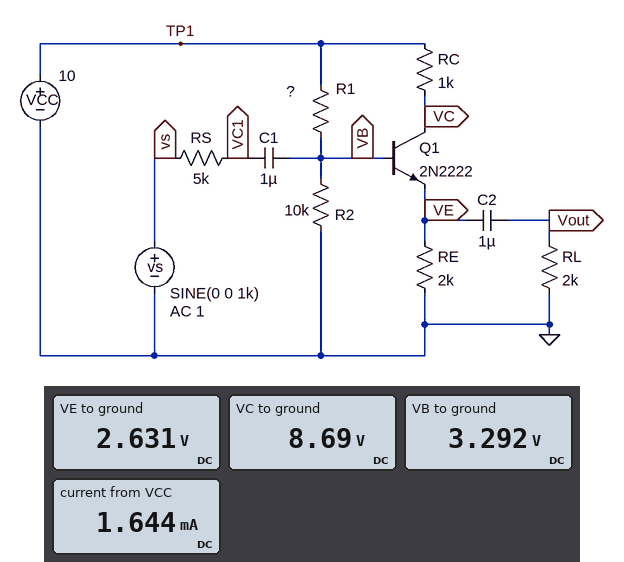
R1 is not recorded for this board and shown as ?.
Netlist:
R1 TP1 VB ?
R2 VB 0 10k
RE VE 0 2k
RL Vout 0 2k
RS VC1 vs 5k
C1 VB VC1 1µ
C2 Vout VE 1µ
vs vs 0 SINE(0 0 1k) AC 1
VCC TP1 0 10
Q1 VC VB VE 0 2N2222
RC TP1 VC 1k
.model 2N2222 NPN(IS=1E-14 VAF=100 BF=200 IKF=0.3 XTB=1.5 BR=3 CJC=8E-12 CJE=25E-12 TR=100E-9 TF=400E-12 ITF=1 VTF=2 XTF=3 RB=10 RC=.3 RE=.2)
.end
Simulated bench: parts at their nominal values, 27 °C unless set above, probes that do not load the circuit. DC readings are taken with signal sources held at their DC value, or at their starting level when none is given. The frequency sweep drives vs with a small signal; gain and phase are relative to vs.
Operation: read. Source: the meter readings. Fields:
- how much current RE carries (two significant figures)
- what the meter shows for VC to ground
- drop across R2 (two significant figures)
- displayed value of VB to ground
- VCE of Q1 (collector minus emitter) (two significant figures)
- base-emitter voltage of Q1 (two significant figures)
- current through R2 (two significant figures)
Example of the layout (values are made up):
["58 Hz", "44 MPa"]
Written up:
["1.3 mA", "8.69 V", "3.3 V", "3.292 V", "6.1 V", "660 mV", "330 µA"]
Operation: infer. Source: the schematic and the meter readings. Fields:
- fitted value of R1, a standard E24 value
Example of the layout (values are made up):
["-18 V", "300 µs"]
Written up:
["20 kΩ"]
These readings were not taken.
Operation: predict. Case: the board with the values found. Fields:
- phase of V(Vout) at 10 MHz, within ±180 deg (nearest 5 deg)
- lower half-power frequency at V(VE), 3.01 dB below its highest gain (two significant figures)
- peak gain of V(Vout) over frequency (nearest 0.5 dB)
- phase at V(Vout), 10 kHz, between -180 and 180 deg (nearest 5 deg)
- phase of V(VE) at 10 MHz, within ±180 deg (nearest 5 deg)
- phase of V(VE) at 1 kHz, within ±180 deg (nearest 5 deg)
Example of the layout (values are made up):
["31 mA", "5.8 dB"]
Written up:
["-45 deg", "13 Hz", "-5.0 dB", "0 deg", "-45 deg", "0 deg"]
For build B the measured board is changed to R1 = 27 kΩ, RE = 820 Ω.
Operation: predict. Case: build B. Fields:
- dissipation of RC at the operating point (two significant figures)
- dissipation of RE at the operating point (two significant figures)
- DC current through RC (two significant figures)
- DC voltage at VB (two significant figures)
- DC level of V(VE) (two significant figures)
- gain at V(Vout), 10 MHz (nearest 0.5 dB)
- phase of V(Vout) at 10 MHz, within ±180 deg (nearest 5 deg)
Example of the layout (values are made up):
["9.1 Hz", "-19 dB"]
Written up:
["5.6 mW", "4.6 mW", "2.4 mA", "2.6 V", "1.9 V", "-13.5 dB", "-55 deg"]
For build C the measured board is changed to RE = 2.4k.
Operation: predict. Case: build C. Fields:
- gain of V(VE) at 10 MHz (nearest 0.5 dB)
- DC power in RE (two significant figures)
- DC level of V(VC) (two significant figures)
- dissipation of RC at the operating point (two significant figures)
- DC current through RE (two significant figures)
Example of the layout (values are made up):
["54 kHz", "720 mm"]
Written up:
["-11.0 dB", "2.9 mW", "8.9 V", "1.2 mW", "1.1 mA"]
